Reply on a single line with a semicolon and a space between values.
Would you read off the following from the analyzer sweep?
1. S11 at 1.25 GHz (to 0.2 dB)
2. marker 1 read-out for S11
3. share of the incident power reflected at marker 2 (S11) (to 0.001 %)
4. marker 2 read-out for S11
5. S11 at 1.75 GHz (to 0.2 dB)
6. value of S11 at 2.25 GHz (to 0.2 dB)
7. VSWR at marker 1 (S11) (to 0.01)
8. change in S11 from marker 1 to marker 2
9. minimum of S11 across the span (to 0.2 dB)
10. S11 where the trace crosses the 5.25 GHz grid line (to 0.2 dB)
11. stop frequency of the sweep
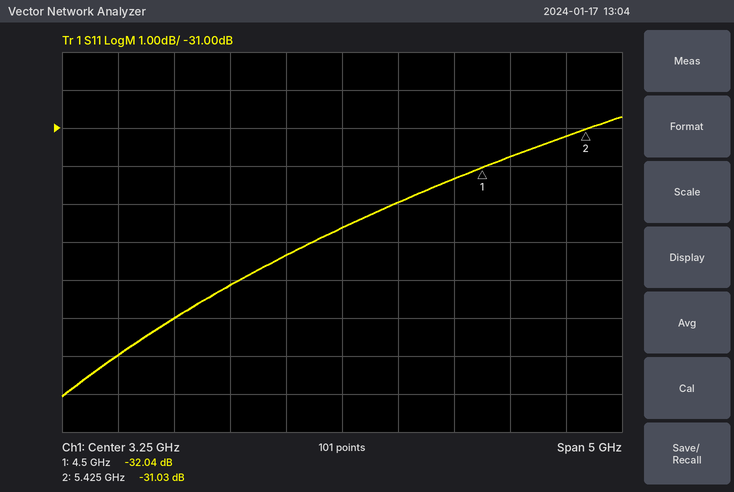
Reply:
-37.0 dB; -32.04 dB; 0.079 %; -31.03 dB; -36.0 dB; -35.2 dB; 1.05; 1.01 dB; -38.0 dB; -31.2 dB; 5.75 GHz
